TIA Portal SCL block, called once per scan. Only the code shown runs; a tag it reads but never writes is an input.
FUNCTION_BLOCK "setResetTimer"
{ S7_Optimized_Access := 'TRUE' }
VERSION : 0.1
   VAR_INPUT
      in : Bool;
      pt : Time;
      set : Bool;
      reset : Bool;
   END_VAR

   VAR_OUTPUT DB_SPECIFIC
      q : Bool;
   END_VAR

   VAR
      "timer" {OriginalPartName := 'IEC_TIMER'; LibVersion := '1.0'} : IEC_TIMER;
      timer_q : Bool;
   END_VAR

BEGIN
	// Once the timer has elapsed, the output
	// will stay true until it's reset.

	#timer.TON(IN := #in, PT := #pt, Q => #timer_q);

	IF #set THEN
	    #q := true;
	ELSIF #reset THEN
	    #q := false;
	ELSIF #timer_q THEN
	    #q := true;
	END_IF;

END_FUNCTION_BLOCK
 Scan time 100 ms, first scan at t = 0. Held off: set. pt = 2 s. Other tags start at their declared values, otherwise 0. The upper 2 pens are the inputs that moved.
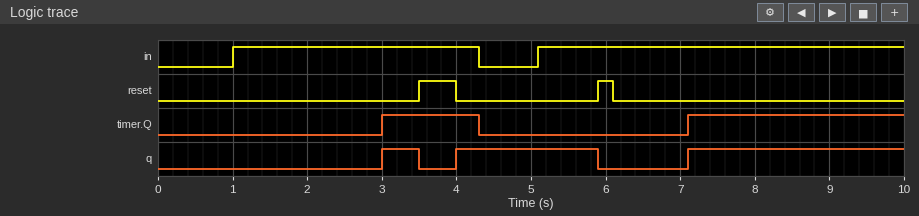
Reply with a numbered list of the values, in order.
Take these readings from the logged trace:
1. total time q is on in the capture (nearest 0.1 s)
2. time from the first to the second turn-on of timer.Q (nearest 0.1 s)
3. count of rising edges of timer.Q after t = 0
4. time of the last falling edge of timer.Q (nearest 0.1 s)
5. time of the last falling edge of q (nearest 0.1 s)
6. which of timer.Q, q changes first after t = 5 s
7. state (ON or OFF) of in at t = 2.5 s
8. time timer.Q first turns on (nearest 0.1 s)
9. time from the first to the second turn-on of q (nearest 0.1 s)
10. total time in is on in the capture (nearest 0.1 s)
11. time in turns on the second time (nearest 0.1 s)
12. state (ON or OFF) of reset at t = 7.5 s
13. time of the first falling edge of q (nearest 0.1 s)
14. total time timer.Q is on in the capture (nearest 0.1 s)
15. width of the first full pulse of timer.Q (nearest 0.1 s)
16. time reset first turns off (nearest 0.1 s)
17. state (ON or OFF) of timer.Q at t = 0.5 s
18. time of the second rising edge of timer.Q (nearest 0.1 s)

1. 5.3 s
2. 4.1 s
3. 2
4. 4.3 s
5. 5.9 s
6. q
7. ON
8. 3.0 s
9. 1.0 s
10. 8.2 s
11. 5.1 s
12. OFF
13. 3.5 s
14. 4.2 s
15. 1.3 s
16. 4.0 s
17. OFF
18. 7.1 s
